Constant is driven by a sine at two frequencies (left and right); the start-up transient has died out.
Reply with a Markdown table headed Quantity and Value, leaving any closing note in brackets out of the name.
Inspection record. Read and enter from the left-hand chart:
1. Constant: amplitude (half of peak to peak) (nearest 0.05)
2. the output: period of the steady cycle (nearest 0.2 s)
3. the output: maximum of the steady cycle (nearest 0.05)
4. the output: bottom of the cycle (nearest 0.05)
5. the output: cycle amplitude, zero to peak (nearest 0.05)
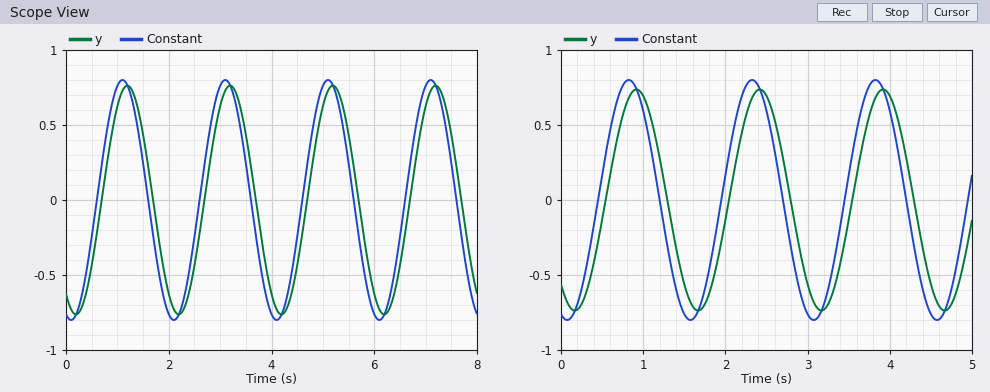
| Quantity | Value |
|---|---|
| Constant: amplitude (half of peak to peak) | 0.80 |
| the output: period of the steady cycle | 2.0 s |
| the output: maximum of the steady cycle | 0.75 |
| the output: bottom of the cycle | -0.75 |
| the output: cycle amplitude, zero to peak | 0.75 |
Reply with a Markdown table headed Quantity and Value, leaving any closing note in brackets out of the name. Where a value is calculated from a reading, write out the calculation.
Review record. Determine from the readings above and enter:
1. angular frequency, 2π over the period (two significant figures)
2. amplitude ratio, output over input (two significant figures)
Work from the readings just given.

| Quantity | Value |
|---|---|
| angular frequency, 2π over the period | 2π / 2 = 3.1 rad/s |
| amplitude ratio, output over input | 0.75 / 0.8 = 0.94 |
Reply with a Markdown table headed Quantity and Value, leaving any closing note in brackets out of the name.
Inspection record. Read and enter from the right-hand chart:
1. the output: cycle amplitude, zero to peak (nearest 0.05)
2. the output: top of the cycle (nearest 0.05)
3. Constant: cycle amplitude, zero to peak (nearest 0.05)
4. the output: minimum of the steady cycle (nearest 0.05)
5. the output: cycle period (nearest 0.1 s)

| Quantity | Value |
|---|---|
| the output: cycle amplitude, zero to peak | 0.75 |
| the output: top of the cycle | 0.75 |
| Constant: cycle amplitude, zero to peak | 0.80 |
| the output: minimum of the steady cycle | -0.75 |
| the output: cycle period | 1.5 s |
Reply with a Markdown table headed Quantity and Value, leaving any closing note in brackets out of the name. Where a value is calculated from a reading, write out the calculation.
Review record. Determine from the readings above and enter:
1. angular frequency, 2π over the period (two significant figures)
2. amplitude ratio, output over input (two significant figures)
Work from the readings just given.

| Quantity | Value |
|---|---|
| angular frequency, 2π over the period | 2π / 1.5 = 4.2 rad/s |
| amplitude ratio, output over input | 0.75 / 0.8 = 0.94 |
